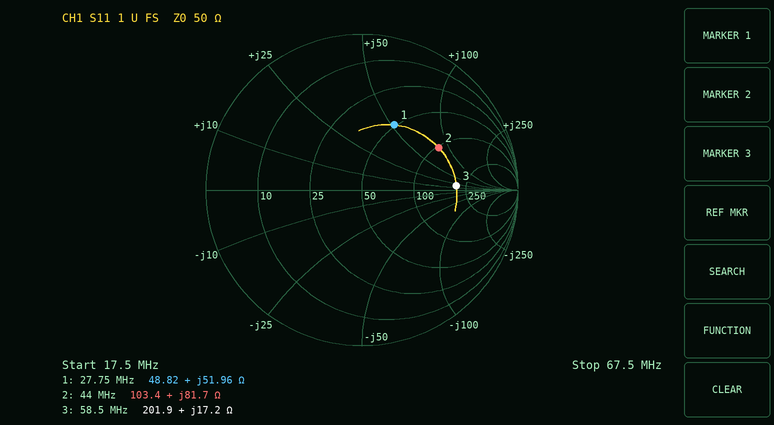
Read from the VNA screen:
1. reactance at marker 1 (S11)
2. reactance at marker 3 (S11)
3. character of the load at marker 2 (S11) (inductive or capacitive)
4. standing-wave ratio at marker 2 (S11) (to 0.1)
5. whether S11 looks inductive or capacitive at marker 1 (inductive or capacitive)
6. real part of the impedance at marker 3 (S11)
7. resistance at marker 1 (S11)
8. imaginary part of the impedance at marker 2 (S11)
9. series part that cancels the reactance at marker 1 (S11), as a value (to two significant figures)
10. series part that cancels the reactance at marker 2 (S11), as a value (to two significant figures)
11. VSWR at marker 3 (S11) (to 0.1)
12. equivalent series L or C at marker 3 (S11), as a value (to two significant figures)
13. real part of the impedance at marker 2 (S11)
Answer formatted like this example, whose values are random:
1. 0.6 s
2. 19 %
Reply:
1. +51.96 Ω
2. +17.2 Ω
3. inductive
4. 3.6
5. inductive
6. 201.9 Ω
7. 48.82 Ω
8. +81.7 Ω
9. 110 pF
10. 44 pF
11. 4.1
12. 47 nH
13. 103.4 Ω
